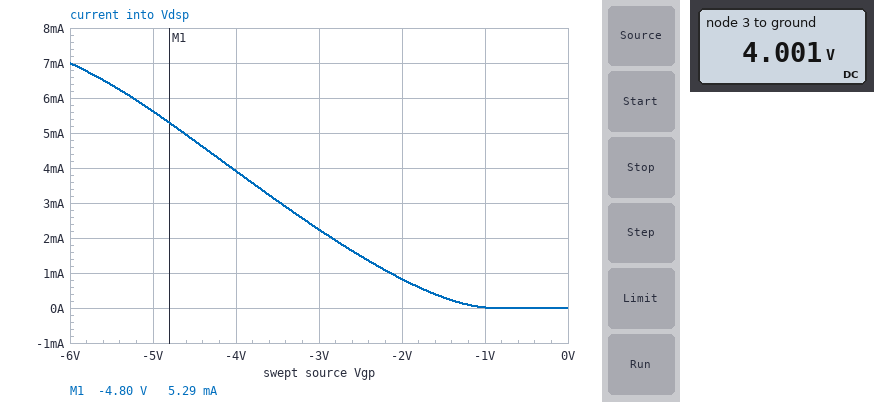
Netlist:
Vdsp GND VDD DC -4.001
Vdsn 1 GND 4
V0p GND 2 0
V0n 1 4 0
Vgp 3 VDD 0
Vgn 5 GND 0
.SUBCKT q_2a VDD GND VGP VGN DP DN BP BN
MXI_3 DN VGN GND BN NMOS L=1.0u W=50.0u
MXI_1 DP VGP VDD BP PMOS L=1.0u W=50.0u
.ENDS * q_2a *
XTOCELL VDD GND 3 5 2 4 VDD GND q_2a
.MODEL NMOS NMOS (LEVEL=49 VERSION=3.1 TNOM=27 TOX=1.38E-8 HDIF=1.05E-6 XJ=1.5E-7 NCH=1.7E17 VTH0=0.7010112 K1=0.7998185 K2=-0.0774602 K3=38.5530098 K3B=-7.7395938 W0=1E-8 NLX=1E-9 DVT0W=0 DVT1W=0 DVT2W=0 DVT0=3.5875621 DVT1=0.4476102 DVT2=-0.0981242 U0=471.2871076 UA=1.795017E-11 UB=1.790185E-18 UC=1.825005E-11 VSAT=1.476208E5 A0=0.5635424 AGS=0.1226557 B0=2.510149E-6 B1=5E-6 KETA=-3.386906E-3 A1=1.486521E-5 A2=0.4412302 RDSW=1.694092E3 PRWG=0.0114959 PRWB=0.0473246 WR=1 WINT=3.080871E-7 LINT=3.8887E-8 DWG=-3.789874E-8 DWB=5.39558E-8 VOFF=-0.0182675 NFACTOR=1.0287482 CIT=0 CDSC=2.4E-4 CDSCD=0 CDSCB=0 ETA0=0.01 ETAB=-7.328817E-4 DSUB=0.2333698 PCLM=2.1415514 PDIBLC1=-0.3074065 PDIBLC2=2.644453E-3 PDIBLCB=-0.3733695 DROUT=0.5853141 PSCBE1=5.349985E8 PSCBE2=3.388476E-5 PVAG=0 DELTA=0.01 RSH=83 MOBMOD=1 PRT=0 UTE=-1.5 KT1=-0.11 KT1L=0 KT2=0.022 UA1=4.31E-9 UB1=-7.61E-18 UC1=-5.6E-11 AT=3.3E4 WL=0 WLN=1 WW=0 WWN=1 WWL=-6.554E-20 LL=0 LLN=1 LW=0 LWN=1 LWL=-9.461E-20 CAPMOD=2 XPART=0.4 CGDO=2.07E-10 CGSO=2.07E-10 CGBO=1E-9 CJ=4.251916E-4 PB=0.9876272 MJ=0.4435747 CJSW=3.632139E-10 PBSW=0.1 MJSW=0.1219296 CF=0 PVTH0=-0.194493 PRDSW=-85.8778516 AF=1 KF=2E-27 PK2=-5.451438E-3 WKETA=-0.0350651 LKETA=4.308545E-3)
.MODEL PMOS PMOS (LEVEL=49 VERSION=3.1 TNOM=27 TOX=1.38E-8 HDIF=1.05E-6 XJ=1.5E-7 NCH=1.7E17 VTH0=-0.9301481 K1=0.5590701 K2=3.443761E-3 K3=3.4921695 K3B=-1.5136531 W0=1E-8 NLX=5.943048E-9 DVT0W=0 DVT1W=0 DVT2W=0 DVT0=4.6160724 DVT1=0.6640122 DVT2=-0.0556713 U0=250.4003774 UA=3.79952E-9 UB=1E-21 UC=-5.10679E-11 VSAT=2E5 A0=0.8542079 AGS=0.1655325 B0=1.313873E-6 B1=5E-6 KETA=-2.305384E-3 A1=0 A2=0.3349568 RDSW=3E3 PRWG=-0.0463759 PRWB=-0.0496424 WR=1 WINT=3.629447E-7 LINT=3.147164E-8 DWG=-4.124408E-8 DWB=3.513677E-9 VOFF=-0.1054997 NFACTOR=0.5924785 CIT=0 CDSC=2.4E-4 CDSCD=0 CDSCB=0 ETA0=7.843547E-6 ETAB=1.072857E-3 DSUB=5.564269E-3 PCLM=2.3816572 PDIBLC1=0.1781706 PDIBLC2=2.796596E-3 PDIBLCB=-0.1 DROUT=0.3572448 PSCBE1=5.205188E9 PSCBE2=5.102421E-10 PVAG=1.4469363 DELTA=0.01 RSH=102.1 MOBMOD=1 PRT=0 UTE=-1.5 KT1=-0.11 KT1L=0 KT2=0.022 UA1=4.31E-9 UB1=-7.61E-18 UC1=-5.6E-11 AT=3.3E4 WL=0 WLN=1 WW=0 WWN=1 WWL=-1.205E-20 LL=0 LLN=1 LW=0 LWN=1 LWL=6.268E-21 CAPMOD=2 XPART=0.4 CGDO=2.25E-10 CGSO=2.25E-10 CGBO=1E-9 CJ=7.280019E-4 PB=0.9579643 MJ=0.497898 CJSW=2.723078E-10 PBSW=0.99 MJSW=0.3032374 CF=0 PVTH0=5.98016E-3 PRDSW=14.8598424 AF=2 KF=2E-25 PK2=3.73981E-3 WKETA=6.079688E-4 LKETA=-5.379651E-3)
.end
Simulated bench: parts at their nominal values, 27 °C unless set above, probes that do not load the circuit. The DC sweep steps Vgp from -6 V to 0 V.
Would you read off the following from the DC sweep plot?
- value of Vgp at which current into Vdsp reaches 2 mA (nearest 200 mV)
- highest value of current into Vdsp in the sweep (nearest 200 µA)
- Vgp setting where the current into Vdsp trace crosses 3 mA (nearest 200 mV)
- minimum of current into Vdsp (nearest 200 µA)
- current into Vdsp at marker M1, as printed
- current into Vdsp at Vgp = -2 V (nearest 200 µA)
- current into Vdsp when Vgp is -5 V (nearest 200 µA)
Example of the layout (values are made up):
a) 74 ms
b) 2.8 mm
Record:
a) -2.8 V
b) 7.0 mA
c) -3.4 V
d) 0 A
e) 5.29 mA
f) 800 µA
g) 5.6 mA
